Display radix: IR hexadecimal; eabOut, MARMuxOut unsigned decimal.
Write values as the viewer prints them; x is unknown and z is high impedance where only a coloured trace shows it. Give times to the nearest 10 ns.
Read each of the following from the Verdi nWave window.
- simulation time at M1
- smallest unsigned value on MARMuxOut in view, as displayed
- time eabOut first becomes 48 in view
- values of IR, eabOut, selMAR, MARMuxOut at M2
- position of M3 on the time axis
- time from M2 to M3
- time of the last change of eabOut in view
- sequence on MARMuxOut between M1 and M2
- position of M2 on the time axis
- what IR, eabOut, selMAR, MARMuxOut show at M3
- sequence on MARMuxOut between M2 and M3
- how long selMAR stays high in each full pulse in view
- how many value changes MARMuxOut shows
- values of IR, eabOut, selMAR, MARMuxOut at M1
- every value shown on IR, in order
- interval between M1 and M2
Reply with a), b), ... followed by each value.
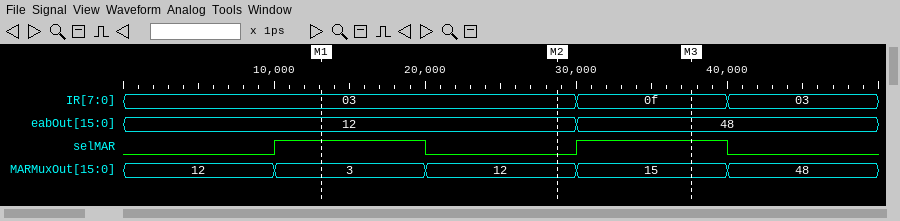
a) 10 ns
b) 3
c) 30 ns
d) IR=03, eabOut=12, selMAR=0, MARMuxOut=12
e) 40 ns
f) 10 ns
g) 30 ns
h) 3, 12
i) 30 ns
j) IR=0f, eabOut=48, selMAR=1, MARMuxOut=15
k) 12, 15
l) 10 ns, 10 ns
m) 4
n) IR=03, eabOut=12, selMAR=1, MARMuxOut=3
o) 03, 0f, 03
p) 20 ns
